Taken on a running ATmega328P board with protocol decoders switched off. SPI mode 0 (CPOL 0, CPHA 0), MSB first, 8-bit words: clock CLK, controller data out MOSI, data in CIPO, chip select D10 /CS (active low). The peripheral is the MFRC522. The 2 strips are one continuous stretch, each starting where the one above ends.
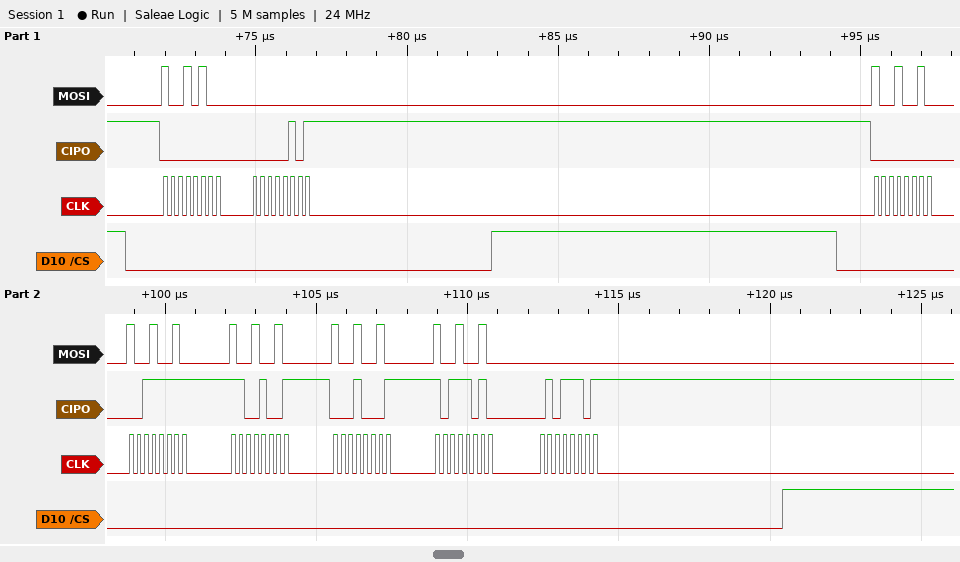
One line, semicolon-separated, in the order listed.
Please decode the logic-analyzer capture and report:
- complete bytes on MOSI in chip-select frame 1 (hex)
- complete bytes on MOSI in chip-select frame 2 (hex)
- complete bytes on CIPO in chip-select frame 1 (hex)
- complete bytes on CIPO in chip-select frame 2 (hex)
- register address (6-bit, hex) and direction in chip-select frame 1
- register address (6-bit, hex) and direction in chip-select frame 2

94 00; 92 92 92 92 92 00; 00 05; 00 3F C9 11 BA 5D; 0x0A read; 0x09 read
